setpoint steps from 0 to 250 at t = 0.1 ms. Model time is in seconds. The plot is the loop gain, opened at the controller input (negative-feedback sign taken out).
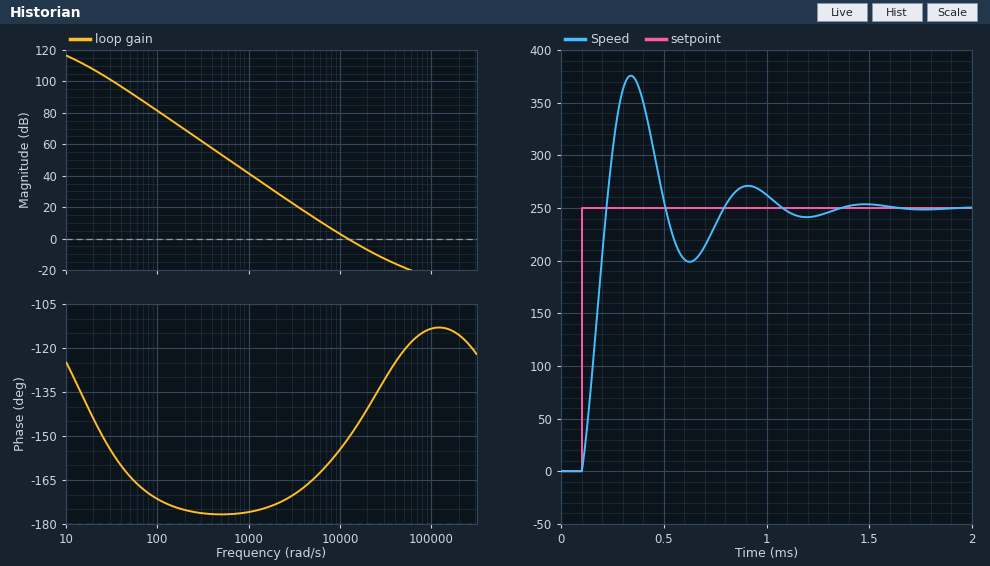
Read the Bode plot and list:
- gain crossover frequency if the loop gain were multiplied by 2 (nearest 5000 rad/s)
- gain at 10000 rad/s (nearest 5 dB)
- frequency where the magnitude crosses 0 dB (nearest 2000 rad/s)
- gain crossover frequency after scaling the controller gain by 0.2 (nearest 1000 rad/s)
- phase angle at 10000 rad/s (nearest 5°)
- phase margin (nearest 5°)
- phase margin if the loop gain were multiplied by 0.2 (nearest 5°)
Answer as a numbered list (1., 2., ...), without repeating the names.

1. 20000 rad/s
2. 5 dB
3. 12000 rad/s
4. 5000 rad/s
5. -155°
6. 30°
7. 15°
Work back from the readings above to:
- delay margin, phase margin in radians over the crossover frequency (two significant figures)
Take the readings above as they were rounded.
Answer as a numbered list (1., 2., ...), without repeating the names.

1. 0.000044 s
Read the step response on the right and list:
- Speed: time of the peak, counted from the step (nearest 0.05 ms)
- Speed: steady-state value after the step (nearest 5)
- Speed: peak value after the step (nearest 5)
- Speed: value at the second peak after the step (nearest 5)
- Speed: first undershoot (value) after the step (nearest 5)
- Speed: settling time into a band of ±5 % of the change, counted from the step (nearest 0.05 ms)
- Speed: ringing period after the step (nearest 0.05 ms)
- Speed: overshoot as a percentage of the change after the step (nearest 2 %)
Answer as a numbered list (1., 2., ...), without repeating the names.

1. 0.25 ms
2. 250
3. 375
4. 270
5. 200
6. 0.90 ms
7. 0.55 ms
8. 50 %
